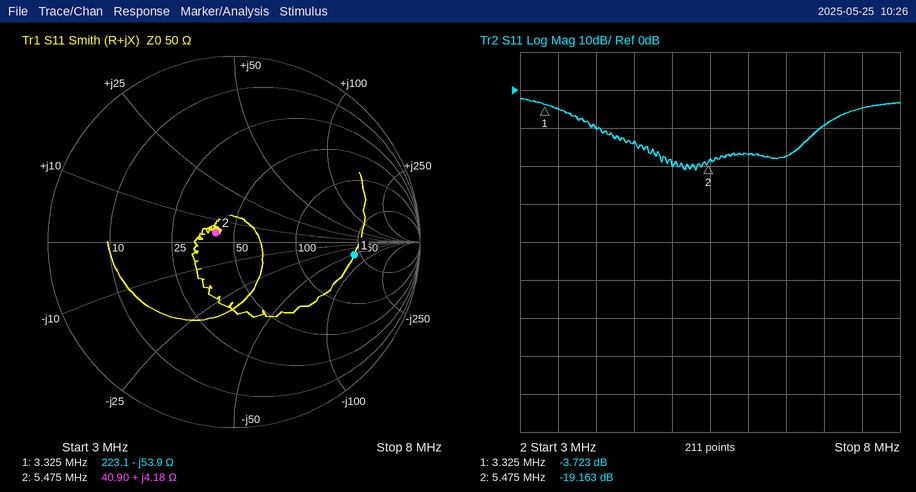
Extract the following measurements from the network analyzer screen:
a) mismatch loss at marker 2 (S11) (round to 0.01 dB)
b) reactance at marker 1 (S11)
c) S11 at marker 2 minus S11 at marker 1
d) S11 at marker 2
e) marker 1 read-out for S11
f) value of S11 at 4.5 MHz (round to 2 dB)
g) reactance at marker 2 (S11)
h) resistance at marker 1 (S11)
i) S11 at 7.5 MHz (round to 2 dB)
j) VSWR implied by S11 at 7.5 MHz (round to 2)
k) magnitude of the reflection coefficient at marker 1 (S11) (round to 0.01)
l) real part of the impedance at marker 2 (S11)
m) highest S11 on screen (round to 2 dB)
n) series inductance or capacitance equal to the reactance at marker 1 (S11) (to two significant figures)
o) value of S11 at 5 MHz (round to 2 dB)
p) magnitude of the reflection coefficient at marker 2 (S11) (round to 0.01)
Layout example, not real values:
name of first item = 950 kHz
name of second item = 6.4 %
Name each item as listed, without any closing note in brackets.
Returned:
mismatch loss at marker 2 (S11) = 0.05 dB
reactance at marker 1 = -53.9 Ω
S11 at marker 2 minus S11 at marker 1 = -15.440 dB
S11 at marker 2 = -19.163 dB
marker 1 read-out for S11 = -3.723 dB
value of S11 at 4.5 MHz = -14 dB
reactance at marker 2 = +4.18 Ω
resistance at marker 1 = 223.1 Ω
S11 at 7.5 MHz = -4 dB
VSWR implied by S11 at 7.5 MHz = 4
magnitude of the reflection coefficient at marker 1 (S11) = 0.65
real part of the impedance at marker 2 = 40.90 Ω
highest S11 on screen = -2 dB
series inductance or capacitance equal to the reactance at marker 1 (S11) = 890 pF
value of S11 at 5 MHz = -20 dB
magnitude of the reflection coefficient at marker 2 (S11) = 0.11
